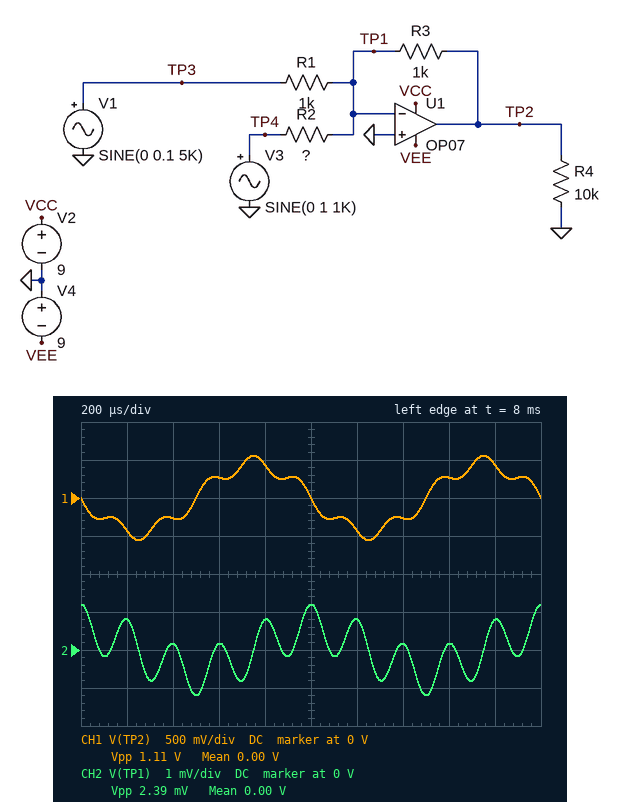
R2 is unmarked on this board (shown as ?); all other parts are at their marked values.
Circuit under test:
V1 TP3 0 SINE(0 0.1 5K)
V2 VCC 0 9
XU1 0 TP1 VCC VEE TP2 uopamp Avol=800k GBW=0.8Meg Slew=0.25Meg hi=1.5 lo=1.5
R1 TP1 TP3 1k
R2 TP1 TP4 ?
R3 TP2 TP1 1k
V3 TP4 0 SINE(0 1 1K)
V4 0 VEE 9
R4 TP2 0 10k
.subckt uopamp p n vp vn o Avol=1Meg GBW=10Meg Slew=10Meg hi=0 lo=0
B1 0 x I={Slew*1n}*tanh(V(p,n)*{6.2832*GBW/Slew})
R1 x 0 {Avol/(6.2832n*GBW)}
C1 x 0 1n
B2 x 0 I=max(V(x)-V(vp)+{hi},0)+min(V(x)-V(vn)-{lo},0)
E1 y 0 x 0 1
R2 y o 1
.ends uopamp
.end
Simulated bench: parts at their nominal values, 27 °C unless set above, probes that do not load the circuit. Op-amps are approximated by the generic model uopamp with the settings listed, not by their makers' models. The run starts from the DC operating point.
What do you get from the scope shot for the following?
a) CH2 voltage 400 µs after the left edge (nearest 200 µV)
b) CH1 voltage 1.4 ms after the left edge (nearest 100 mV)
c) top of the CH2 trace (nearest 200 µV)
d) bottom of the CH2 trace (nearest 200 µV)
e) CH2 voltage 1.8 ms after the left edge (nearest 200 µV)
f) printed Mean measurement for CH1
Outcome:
200 µV
-300 mV
1.2 mV
-1.2 mV
800 µV
0.00 V
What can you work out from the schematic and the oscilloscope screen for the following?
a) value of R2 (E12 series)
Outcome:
2.2 kΩ
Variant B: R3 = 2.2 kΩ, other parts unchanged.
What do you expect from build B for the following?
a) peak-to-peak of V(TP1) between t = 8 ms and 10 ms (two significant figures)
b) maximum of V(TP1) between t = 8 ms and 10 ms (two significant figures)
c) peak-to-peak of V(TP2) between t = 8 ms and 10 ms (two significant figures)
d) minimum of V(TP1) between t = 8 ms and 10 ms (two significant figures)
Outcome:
5.3 mV
2.6 mV
2.4 V
-2.6 mV
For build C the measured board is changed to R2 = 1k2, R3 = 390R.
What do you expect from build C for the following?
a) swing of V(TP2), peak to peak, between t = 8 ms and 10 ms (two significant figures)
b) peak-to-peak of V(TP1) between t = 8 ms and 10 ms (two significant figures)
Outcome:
730 mV
1.3 mV
